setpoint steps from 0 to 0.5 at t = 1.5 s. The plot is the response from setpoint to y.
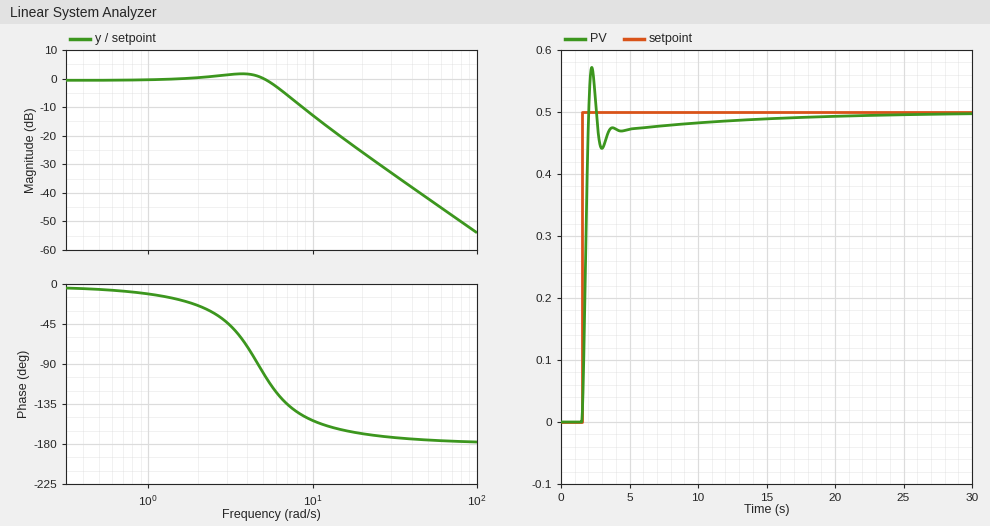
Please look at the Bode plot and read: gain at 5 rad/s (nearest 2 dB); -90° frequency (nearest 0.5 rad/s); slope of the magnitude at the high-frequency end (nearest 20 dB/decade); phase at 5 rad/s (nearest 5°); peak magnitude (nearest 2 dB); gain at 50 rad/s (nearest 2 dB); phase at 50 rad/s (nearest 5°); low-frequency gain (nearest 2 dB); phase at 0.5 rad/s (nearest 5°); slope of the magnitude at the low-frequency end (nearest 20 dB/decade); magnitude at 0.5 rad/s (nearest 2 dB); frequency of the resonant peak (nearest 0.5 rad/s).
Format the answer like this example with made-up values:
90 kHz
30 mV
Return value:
0 dB
4.5 rad/s
-40 dB/decade
-100°
2 dB
-42 dB
-175°
0 dB
-5°
0 dB/decade
0 dB
3.5 rad/s
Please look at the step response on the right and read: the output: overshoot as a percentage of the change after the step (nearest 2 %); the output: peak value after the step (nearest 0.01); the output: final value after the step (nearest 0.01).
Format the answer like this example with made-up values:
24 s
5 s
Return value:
14 %
0.57
0.50
